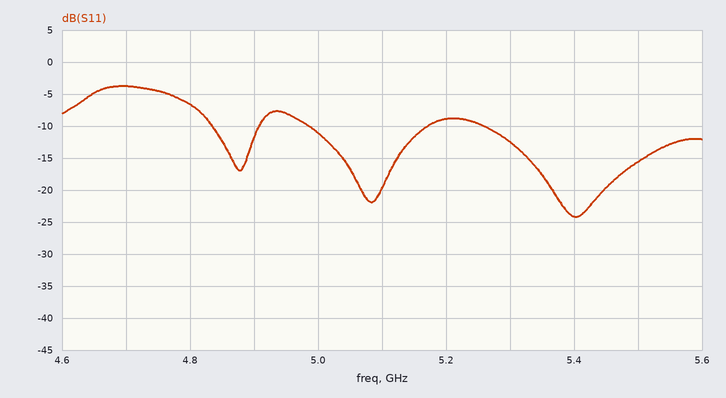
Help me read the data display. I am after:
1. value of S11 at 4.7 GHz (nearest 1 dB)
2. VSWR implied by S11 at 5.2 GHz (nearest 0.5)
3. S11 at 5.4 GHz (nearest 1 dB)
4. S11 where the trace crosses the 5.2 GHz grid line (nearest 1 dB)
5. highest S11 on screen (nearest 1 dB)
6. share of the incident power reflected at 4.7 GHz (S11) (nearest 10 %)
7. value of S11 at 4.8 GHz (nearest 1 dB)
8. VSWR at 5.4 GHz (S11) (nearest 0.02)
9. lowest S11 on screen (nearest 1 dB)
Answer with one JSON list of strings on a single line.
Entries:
["-4 dB", "2.0", "-24 dB", "-9 dB", "-4 dB", "40 %", "-7 dB", "1.14", "-24 dB"]
